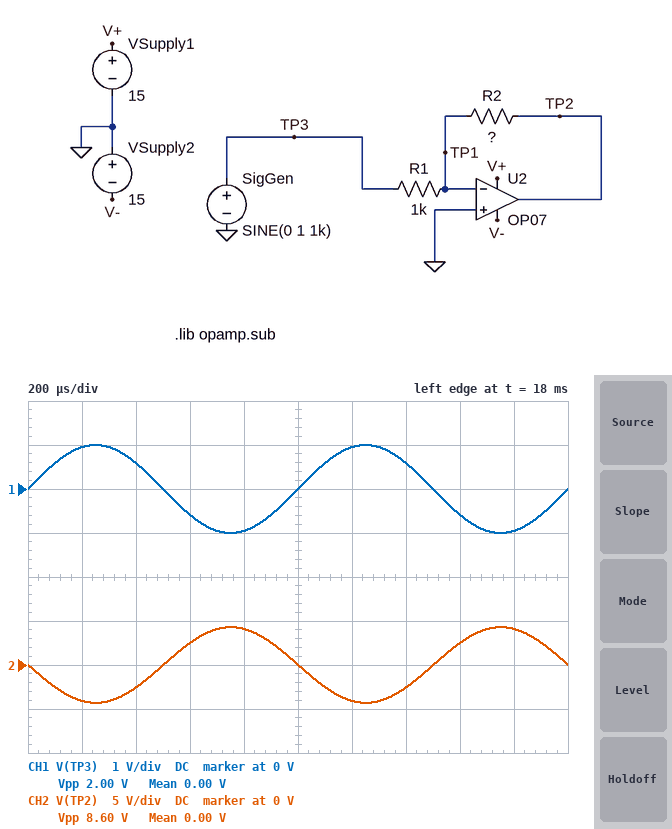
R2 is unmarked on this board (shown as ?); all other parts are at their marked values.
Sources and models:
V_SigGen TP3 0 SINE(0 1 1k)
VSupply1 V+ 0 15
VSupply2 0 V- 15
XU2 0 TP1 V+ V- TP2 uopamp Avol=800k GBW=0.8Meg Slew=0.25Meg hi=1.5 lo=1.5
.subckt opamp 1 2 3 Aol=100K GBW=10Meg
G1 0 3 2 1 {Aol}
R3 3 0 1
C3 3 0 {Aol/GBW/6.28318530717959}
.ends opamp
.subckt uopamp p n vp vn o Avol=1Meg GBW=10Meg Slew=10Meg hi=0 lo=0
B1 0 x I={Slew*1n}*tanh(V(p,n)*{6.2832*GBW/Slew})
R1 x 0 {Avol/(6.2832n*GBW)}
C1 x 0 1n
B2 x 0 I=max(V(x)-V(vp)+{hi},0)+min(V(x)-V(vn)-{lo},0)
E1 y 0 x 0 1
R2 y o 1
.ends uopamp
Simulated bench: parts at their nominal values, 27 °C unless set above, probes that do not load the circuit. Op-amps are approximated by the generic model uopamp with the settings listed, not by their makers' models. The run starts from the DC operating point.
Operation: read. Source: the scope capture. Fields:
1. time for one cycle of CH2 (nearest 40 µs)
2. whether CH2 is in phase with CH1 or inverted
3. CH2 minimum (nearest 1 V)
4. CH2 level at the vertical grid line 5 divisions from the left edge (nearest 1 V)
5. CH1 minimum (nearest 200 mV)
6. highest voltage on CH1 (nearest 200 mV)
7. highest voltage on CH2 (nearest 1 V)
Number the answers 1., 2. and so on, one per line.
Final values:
1. 1.00 ms
2. inverted
3. -4 V
4. 0 V
5. -1.0 V
6. 1.0 V
7. 4 V
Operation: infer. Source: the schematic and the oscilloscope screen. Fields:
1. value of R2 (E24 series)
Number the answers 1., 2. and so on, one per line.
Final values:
1. 4.3 kΩ
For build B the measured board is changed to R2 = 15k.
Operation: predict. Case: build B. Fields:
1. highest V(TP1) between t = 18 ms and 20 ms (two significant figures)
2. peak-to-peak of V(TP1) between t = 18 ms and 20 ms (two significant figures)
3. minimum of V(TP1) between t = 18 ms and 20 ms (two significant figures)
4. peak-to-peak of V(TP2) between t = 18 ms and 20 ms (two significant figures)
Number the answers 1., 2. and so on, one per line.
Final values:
1. 94 mV
2. 190 mV
3. -94 mV
4. 27 V
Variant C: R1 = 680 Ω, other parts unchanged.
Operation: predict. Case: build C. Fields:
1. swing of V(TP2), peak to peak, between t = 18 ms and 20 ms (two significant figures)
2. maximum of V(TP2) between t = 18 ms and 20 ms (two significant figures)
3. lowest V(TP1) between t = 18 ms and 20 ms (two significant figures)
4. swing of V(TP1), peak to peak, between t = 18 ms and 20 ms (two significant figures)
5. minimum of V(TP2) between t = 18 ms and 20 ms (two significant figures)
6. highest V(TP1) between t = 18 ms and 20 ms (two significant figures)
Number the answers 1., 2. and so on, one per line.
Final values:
1. 13 V
2. 6.3 V
3. -8.0 mV
4. 16 mV
5. -6.3 V
6. 8.0 mV
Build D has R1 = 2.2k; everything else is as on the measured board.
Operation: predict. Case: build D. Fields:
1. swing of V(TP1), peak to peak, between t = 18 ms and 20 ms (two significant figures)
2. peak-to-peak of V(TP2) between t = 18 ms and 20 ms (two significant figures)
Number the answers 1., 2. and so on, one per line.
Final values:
1. 4.9 mV
2. 3.9 V
